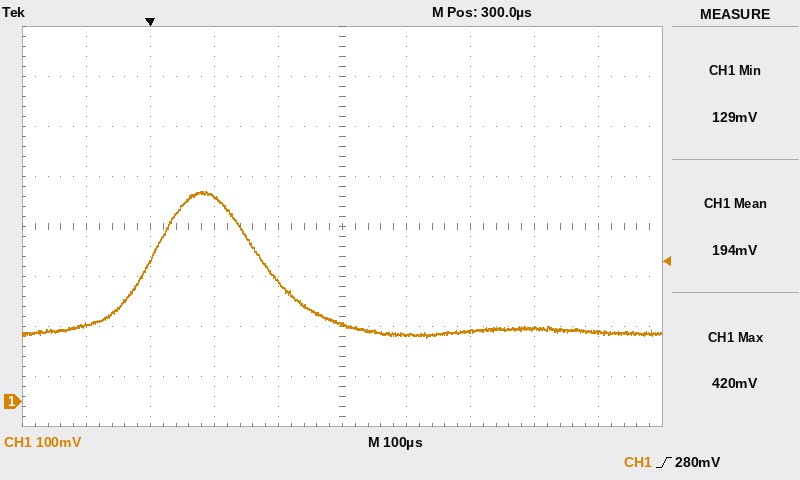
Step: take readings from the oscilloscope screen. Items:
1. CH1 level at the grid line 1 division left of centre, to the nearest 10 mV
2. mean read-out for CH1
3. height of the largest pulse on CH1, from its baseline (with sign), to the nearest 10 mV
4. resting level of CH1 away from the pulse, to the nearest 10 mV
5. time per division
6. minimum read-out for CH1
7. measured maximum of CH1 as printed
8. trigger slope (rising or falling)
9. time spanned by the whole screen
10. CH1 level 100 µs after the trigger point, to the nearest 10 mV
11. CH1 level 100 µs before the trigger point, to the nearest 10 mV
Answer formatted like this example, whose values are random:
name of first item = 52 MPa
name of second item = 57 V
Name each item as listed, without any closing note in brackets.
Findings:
CH1 level at the grid line 1 division left of centre, to the nearest 10 mV = 240 mV
mean read-out for CH1 = 194 mV
height of the largest pulse on CH1, from its baseline (with sign), to the nearest 10 mV = +280 mV
resting level of CH1 away from the pulse, to the nearest 10 mV = 140 mV
time per division = 100 µs
minimum read-out for CH1 = 129 mV
measured maximum of CH1 as printed = 420 mV
trigger slope = rising
time spanned by the whole screen = 1 ms
CH1 level 100 µs after the trigger point, to the nearest 10 mV = 410 mV
CH1 level 100 µs before the trigger point, to the nearest 10 mV = 150 mV
